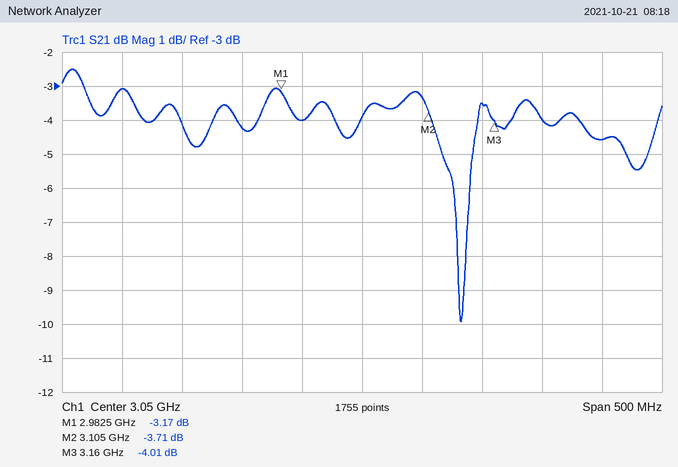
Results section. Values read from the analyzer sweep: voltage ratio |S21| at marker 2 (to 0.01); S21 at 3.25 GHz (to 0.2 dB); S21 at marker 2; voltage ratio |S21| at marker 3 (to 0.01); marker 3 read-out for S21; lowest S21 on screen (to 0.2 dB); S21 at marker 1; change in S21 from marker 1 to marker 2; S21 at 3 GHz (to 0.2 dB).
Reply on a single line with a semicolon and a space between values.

0.65; -4.6 dB; -3.71 dB; 0.63; -4.01 dB; -10.0 dB; -3.17 dB; -0.54 dB; -4.0 dB
